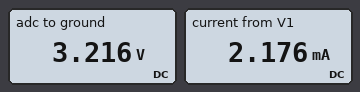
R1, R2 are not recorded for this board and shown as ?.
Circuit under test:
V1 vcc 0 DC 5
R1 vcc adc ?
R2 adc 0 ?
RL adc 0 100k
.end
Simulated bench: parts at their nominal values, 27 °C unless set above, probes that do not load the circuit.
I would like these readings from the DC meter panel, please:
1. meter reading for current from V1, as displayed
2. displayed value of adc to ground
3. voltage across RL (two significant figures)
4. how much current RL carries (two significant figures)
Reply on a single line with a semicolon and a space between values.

2.176 mA; 3.216 V; 3.2 V; 32 µA
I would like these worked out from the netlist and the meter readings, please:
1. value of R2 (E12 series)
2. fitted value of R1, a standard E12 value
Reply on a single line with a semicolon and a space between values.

1.5 kΩ; 820 Ω
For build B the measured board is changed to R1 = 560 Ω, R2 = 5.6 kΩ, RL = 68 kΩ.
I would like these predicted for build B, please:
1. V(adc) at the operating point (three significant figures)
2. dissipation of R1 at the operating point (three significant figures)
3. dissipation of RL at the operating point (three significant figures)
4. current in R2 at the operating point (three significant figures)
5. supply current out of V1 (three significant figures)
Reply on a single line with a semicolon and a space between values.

4.51 V; 426 µW; 299 µW; 806 µA; 872 µA
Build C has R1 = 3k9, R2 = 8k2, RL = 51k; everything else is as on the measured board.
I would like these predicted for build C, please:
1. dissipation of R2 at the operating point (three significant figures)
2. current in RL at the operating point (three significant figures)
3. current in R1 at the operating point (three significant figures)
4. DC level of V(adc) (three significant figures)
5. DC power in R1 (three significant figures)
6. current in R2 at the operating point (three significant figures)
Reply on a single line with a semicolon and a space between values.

1.27 mW; 63.2 µA; 456 µA; 3.22 V; 811 µW; 393 µA
